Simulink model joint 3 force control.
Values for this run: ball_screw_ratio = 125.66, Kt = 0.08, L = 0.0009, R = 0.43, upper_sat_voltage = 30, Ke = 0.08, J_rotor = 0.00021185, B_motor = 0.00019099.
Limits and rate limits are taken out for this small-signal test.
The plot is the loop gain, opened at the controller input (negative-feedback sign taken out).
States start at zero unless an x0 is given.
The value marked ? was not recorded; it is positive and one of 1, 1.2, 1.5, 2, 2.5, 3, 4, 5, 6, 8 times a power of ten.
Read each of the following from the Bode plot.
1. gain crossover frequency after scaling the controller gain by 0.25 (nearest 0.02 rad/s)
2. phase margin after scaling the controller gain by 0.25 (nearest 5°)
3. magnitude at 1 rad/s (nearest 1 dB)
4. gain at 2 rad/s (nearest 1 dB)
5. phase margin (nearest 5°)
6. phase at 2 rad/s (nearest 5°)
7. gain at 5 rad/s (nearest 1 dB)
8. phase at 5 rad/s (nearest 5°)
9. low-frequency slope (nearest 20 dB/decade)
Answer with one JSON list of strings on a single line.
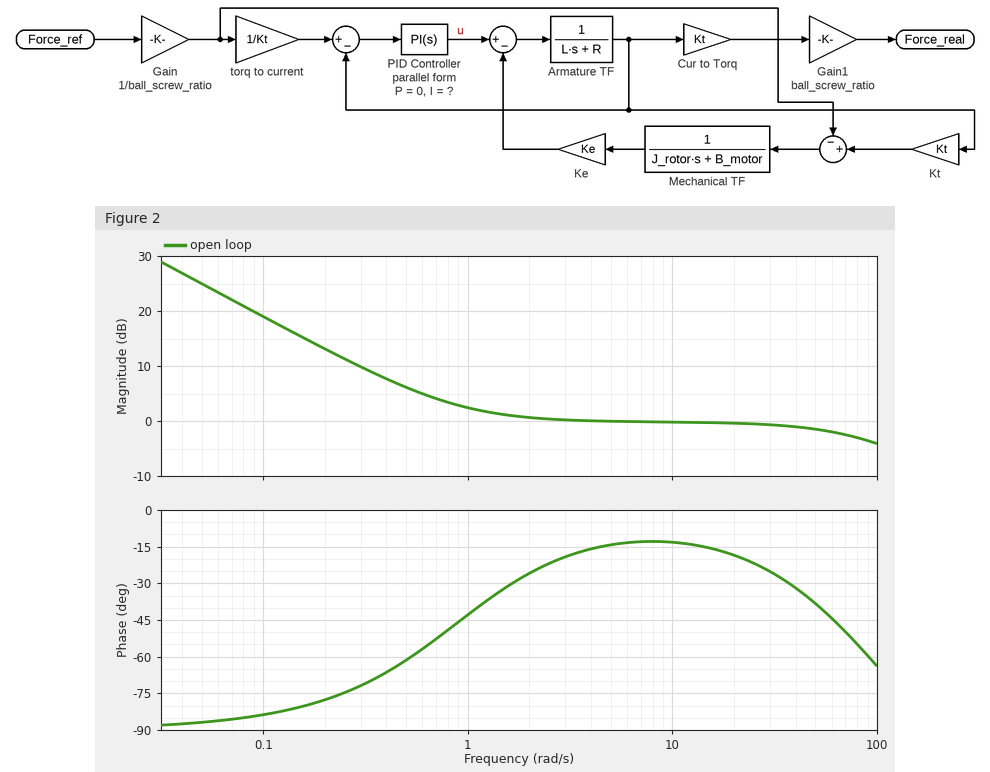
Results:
["0.22 rad/s", "105°", "2 dB", "1 dB", "165°", "-25°", "0 dB", "-15°", "-20 dB/decade"]
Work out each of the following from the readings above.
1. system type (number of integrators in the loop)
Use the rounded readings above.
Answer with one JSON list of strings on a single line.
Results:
["1"]
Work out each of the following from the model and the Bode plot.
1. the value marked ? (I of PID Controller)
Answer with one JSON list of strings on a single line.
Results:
["30"]
